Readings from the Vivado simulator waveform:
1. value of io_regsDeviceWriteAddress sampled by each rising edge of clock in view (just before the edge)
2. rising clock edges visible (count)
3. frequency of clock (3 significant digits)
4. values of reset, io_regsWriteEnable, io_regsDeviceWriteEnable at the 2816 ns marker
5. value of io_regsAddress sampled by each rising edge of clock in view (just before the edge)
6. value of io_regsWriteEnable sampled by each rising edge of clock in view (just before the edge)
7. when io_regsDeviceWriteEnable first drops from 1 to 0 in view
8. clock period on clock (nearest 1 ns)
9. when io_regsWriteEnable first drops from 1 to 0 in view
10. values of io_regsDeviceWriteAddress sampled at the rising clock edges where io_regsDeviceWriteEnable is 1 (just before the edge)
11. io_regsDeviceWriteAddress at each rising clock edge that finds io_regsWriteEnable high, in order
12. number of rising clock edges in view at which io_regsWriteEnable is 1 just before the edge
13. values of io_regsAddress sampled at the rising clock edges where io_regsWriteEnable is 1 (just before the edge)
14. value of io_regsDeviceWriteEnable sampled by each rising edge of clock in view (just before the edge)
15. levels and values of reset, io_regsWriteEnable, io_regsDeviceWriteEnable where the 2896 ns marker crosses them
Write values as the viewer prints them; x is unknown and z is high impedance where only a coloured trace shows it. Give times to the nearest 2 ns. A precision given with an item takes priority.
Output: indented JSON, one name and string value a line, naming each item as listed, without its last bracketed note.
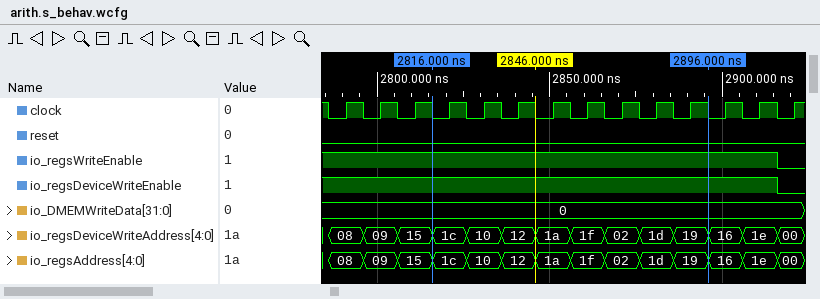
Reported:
{
  "value of io_regsDeviceWriteAddress sampled by each rising edge of clock in view": "08, 09, 15, 1c, 10, 12, 1a, 1f, 02, 1d, 19, 16, 1e, 00",
  "rising clock edges visible": "14",
  "frequency of clock": "100 MHz",
  "values of reset, io_regsWriteEnable, io_regsDeviceWriteEnable at the 2816 ns marker": "reset=0, io_regsWriteEnable=1, io_regsDeviceWriteEnable=1",
  "value of io_regsAddress sampled by each rising edge of clock in view": "08, 09, 15, 1c, 10, 12, 1a, 1f, 02, 1d, 19, 16, 1e, 00",
  "value of io_regsWriteEnable sampled by each rising edge of clock in view": "1 1 1 1 1 1 1 1 1 1 1 1 1 0",
  "when io_regsDeviceWriteEnable first drops from 1 to 0 in view": "2916 ns",
  "clock period on clock": "10 ns",
  "when io_regsWriteEnable first drops from 1 to 0 in view": "2916 ns",
  "values of io_regsDeviceWriteAddress sampled at the rising clock edges where io_regsDeviceWriteEnable is 1": "08, 09, 15, 1c, 10, 12, 1a, 1f, 02, 1d, 19, 16, 1e",
  "io_regsDeviceWriteAddress at each rising clock edge that finds io_regsWriteEnable high, in order": "08, 09, 15, 1c, 10, 12, 1a, 1f, 02, 1d, 19, 16, 1e",
  "number of rising clock edges in view at which io_regsWriteEnable is 1 just before the edge": "13",
  "values of io_regsAddress sampled at the rising clock edges where io_regsWriteEnable is 1": "08, 09, 15, 1c, 10, 12, 1a, 1f, 02, 1d, 19, 16, 1e",
  "value of io_regsDeviceWriteEnable sampled by each rising edge of clock in view": "1 1 1 1 1 1 1 1 1 1 1 1 1 0",
  "levels and values of reset, io_regsWriteEnable, io_regsDeviceWriteEnable where the 2896 ns marker crosses them": "reset=0, io_regsWriteEnable=1, io_regsDeviceWriteEnable=1"
}
